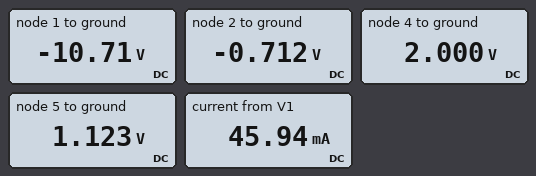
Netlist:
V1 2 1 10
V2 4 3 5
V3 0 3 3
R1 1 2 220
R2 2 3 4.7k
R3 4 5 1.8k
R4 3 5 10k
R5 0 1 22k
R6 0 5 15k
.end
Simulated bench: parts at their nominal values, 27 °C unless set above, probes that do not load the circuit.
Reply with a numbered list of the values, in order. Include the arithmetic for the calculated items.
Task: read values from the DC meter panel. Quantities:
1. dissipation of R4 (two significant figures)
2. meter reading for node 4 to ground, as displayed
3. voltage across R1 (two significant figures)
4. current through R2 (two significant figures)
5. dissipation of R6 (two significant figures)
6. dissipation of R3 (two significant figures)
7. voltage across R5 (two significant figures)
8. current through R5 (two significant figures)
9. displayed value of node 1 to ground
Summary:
1. (1.123 V - (-3 V))^2 / 10 kΩ = 1.7 mW
2. 2.000 V
3. -712 mV - (-10.71 V) = 10 V
4. (-712 mV - (-3 V)) / 4.7 kΩ = 490 µA
5. (1.123 V)^2 / 15 kΩ = 84 µW
6. (2 V - 1.123 V)^2 / 1.8 kΩ = 430 µW
7. 0 V - (-10.71 V) = 11 V
8. (0 V - (-10.71 V)) / 22 kΩ = 490 µA
9. -10.71 V
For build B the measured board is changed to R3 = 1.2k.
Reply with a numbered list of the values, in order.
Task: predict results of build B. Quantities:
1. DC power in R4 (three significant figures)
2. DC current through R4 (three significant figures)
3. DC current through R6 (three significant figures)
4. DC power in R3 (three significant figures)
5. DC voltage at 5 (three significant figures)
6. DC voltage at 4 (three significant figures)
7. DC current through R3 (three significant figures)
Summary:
1. 1.91 mW
2. 437 µA
3. 91.1 µA
4. 334 µW
5. 1.37 V
6. 2.00 V
7. 528 µA
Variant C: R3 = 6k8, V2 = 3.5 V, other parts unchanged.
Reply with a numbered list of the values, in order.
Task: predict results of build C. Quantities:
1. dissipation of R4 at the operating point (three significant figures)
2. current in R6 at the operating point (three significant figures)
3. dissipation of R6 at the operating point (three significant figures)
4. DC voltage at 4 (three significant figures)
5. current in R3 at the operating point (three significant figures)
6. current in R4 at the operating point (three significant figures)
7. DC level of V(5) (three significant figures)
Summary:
1. 519 µW
2. 48.1 µA
3. 34.7 µW
4. 500 mV
5. 180 µA
6. 228 µA
7. -722 mV
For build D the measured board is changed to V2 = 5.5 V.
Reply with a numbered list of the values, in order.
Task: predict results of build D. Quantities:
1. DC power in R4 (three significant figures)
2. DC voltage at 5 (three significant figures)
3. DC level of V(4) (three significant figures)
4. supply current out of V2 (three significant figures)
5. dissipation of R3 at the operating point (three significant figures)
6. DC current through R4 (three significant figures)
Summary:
1. 2.03 mW
2. 1.51 V
3. 2.50 V
4. 551 µA
5. 547 µW
6. 451 µA
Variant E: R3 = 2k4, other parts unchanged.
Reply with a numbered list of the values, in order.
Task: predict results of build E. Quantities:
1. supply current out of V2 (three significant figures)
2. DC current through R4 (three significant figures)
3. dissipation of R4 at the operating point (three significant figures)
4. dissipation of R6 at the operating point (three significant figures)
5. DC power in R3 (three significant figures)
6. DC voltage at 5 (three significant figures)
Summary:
1. 452 µA
2. 391 µA
3. 1.53 mW
4. 55.7 µW
5. 491 µW
6. 914 mV
